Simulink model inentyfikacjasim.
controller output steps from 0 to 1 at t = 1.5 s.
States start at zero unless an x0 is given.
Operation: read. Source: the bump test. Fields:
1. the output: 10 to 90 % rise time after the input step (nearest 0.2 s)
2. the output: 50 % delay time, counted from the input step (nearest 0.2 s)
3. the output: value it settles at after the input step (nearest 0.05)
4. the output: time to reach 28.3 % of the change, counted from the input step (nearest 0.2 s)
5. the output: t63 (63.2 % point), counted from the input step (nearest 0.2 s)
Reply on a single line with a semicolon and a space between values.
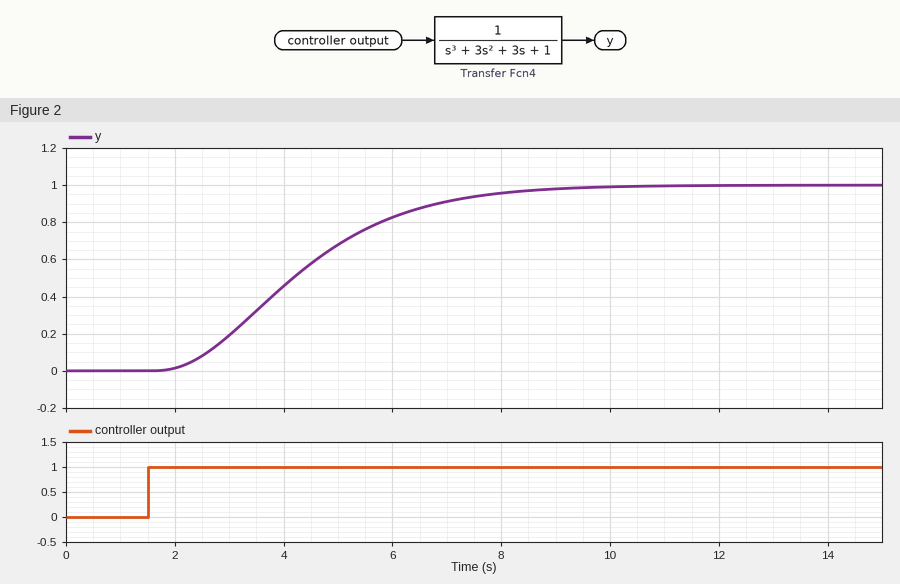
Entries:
4.2 s; 2.6 s; 1.00; 1.8 s; 3.2 s
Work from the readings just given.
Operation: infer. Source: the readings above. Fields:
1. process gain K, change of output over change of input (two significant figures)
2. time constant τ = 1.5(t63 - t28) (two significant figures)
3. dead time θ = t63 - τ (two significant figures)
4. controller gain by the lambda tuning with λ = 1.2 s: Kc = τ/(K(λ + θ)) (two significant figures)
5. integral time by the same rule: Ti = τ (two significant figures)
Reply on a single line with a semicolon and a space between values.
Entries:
1.0; 2.1 s; 1.1 s; 0.91; 2.1 s
